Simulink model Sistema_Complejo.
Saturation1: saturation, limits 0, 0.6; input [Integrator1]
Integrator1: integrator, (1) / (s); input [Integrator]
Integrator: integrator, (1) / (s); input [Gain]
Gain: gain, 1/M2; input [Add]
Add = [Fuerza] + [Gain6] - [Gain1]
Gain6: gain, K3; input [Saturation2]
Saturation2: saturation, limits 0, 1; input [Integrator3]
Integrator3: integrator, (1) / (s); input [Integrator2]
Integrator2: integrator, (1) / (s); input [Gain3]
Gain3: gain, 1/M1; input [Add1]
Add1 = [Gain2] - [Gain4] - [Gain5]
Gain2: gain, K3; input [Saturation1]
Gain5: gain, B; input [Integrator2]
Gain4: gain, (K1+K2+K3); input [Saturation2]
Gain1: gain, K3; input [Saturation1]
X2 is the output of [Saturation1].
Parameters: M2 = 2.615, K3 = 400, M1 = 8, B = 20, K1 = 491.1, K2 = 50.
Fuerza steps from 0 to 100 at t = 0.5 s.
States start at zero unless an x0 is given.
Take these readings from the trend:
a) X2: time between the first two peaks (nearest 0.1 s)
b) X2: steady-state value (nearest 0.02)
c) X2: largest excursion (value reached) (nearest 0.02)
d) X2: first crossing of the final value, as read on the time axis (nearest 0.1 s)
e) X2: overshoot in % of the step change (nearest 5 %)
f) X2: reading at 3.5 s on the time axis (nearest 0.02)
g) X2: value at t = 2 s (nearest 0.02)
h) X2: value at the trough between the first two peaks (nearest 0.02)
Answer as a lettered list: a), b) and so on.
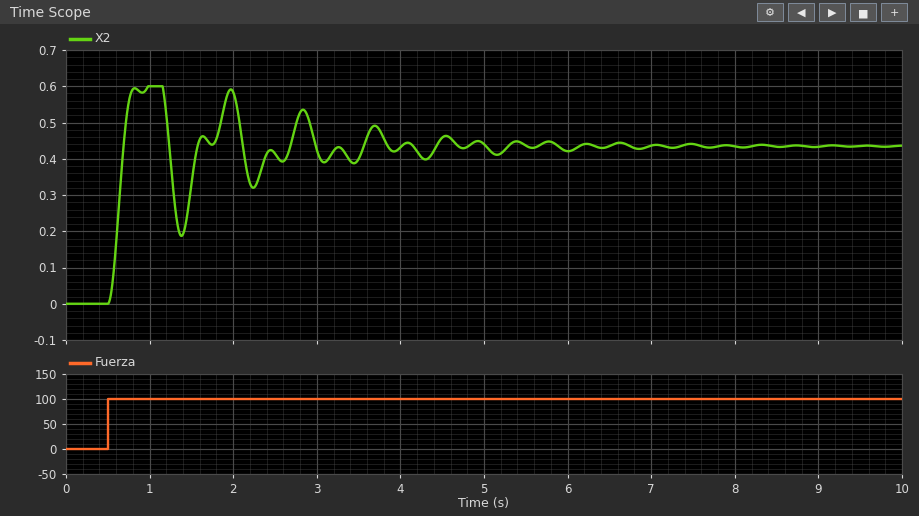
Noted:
a) 0.9 s
b) 0.44
c) 0.60
d) 0.7 s
e) 40 %
f) 0.40
g) 0.58
h) 0.18
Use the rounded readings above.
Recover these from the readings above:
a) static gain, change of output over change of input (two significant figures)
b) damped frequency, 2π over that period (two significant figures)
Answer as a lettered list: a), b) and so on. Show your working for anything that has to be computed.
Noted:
a) (0.44 - 0) / (100 - 0) = 0.0044
b) 2π / 0.9 = 7.0 rad/s
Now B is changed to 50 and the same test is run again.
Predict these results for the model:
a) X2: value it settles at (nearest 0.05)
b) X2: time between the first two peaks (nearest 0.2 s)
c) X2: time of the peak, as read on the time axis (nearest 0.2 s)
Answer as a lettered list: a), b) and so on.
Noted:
a) 0.45
b) 1.2 s
c) 0.8 s
